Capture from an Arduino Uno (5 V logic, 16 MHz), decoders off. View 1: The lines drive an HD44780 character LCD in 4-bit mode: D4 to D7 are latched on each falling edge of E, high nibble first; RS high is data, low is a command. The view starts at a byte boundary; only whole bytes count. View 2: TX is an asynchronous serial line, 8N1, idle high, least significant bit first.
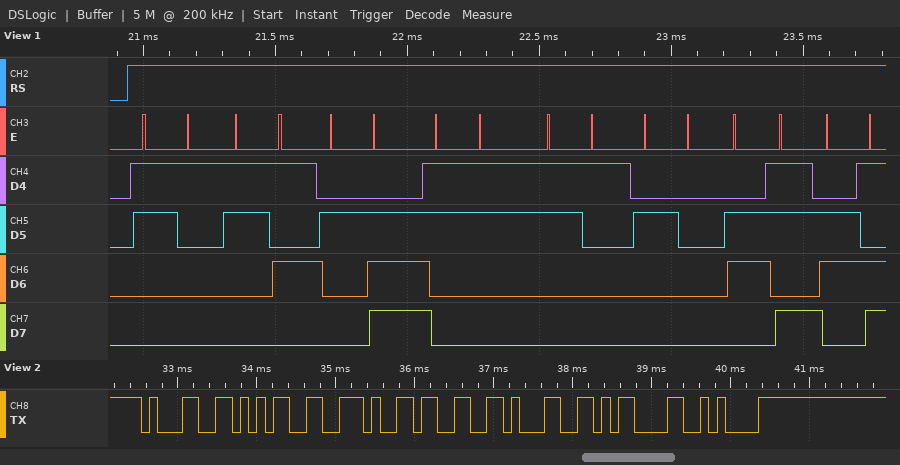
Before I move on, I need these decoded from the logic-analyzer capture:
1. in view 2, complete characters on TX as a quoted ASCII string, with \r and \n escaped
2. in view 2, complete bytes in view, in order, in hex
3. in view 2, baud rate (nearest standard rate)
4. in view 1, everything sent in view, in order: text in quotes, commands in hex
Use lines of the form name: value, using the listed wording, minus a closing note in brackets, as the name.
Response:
in view 2, complete characters on TX as a quoted ASCII string, with \r and \n escaped: "15.31\r\n"
in view 2, complete bytes in view, in order, in hex: 31 35 2E 33 31 0D 0A
in view 2, baud rate: 9600 baud
in view 1, everything sent in view, in order: text in quotes, commands in hex: "15.31 km"
